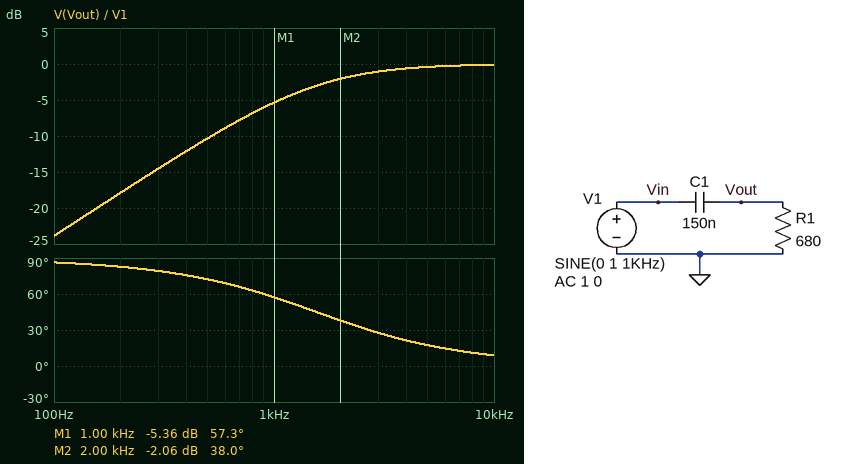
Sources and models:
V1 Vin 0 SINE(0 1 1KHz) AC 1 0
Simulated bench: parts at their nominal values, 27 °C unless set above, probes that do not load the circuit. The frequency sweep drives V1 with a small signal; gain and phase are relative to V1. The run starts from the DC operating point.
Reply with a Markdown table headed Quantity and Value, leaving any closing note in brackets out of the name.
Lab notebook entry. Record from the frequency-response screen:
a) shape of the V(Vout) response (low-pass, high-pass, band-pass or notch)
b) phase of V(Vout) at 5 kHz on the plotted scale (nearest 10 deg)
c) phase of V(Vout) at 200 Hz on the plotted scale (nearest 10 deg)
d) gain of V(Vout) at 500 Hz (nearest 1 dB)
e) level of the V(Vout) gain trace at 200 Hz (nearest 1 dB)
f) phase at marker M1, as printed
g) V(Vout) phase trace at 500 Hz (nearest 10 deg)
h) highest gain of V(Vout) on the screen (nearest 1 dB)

| Quantity | Value |
|---|---|
| shape of the V(Vout) response | high-pass |
| phase of V(Vout) at 5 kHz on the plotted scale | 20 deg |
| phase of V(Vout) at 200 Hz on the plotted scale | 80 deg |
| gain of V(Vout) at 500 Hz | -10 dB |
| level of the V(Vout) gain trace at 200 Hz | -18 dB |
| phase at marker M1, as printed | 57.3 deg |
| V(Vout) phase trace at 500 Hz | 70 deg |
| highest gain of V(Vout) on the screen | 0 dB |
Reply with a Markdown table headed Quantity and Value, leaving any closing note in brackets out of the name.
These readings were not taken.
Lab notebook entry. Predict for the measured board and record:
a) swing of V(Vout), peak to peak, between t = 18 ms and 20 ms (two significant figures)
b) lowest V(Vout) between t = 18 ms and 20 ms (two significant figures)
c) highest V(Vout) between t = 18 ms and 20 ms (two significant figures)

| Quantity | Value |
|---|---|
| swing of V(Vout), peak to peak, between t = 18 ms and 20 ms | 1.1 V |
| lowest V(Vout) between t = 18 ms and 20 ms | -540 mV |
| highest V(Vout) between t = 18 ms and 20 ms | 540 mV |
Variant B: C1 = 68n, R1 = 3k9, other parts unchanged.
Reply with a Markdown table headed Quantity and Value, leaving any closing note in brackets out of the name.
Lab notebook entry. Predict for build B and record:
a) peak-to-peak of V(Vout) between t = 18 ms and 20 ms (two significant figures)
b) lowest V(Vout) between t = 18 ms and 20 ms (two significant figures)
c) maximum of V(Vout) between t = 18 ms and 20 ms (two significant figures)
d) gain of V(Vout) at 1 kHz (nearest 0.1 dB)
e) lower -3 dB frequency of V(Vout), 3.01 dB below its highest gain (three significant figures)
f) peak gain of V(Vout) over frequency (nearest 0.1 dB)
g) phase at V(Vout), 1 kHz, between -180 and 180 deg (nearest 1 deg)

| Quantity | Value |
|---|---|
| peak-to-peak of V(Vout) between t = 18 ms and 20 ms | 1.7 V |
| lowest V(Vout) between t = 18 ms and 20 ms | -860 mV |
| maximum of V(Vout) between t = 18 ms and 20 ms | 860 mV |
| gain of V(Vout) at 1 kHz | -1.3 dB |
| lower -3 dB frequency of V(Vout), 3.01 dB below its highest gain | 600 Hz |
| peak gain of V(Vout) over frequency | 0 dB |
| phase at V(Vout), 1 kHz, between -180 and 180 deg | 31 deg |
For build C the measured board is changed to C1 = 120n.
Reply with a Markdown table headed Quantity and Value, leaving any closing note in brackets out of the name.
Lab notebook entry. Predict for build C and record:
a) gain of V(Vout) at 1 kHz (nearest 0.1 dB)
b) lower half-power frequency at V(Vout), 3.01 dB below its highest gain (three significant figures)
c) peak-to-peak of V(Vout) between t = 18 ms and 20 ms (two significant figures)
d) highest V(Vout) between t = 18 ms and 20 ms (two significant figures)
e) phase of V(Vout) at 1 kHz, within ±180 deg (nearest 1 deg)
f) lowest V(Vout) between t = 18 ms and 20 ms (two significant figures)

| Quantity | Value |
|---|---|
| gain of V(Vout) at 1 kHz | -6.8 dB |
| lower half-power frequency at V(Vout), 3.01 dB below its highest gain | 1.95 kHz |
| peak-to-peak of V(Vout) between t = 18 ms and 20 ms | 910 mV |
| highest V(Vout) between t = 18 ms and 20 ms | 460 mV |
| phase of V(Vout) at 1 kHz, within ±180 deg | 63 deg |
| lowest V(Vout) between t = 18 ms and 20 ms | -460 mV |
